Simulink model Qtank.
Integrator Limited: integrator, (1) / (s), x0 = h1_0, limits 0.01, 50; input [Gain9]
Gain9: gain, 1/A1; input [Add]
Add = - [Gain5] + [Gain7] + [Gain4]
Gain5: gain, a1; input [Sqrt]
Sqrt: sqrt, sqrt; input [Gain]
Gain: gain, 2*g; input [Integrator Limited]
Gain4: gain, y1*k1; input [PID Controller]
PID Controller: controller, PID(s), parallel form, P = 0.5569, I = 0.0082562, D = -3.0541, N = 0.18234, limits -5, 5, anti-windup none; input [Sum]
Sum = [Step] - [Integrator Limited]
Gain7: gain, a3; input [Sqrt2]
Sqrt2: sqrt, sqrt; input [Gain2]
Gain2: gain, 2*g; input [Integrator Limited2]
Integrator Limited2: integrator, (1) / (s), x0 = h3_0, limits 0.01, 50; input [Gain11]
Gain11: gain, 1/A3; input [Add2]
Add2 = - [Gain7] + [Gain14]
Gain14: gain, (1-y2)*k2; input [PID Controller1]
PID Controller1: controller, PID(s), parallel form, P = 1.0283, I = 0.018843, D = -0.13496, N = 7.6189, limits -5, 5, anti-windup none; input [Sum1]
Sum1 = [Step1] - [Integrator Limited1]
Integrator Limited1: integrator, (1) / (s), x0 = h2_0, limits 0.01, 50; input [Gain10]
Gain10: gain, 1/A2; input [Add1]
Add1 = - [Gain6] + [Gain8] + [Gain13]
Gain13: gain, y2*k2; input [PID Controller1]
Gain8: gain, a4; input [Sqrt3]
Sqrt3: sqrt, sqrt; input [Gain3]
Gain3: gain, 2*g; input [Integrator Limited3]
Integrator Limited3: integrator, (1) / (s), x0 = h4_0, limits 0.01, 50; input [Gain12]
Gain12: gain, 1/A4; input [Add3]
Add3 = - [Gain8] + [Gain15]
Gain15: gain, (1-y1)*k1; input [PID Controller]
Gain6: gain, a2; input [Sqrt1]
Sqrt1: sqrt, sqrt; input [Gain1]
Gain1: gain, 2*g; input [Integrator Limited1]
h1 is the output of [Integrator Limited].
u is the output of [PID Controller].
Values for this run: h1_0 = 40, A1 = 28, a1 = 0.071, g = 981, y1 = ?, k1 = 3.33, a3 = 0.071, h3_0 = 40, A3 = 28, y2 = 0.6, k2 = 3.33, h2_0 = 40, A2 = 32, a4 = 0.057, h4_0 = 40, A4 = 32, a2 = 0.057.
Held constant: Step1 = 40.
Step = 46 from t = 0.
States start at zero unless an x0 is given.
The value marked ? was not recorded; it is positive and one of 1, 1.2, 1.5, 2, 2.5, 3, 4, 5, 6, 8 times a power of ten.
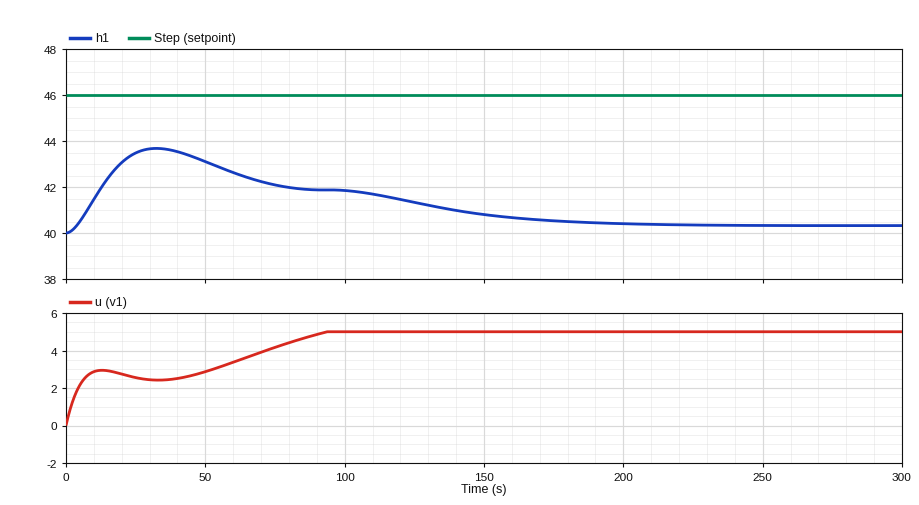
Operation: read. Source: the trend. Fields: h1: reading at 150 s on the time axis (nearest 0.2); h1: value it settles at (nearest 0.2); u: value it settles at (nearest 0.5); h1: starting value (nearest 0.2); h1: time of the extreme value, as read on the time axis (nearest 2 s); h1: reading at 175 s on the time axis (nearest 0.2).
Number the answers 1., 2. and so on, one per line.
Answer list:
1. 40.8
2. 40.4
3. 5.0
4. 40.0
5. 32 s
6. 40.6
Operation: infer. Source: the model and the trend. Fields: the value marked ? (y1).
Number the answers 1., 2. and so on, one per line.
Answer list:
1. 0.8
